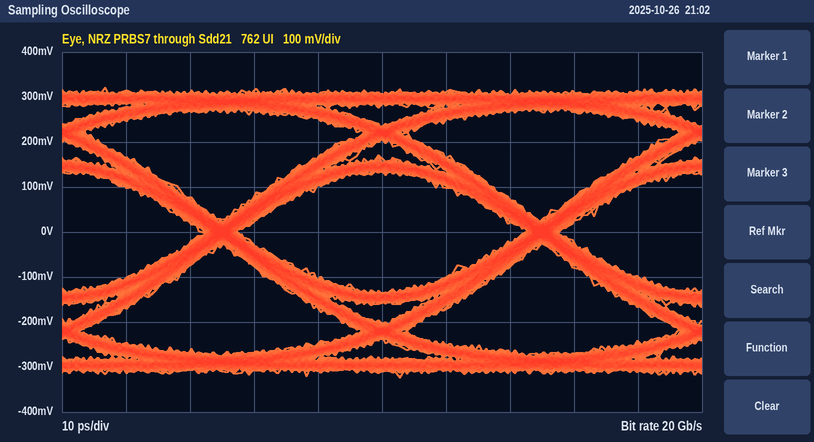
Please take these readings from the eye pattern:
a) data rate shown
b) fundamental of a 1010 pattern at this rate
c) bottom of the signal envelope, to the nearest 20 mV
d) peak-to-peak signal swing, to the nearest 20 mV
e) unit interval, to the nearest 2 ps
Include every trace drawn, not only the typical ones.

20 Gb/s
10 GHz
-320 mV
640 mV
50 ps
